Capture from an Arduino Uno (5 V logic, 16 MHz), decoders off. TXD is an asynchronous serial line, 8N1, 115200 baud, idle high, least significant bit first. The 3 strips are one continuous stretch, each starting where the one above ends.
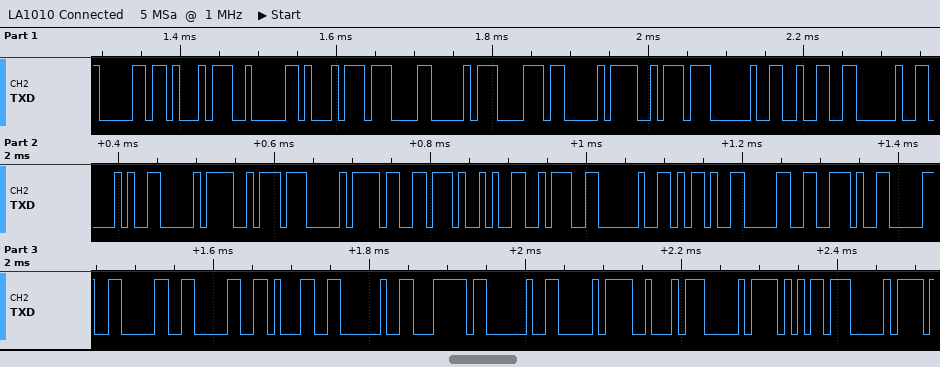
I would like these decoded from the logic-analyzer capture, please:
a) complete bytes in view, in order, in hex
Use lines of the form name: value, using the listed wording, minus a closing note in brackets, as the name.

complete bytes in view, in order, in hex: 0xB0 0xD1 0x82 0xD1 0x87 0xD0 0xB8 0xD0 0xBA 0x20 0x32 0x20 0x28 0xD0 0xBA 0xD0 0xB3 0x29 0x3A 0x20 0x2D 0x30 0x2E 0x30 0x30 0x30 0x31 0x20 0x7C 0x20 0xD0 0xA2 0xD0 0xB5 0xD0
